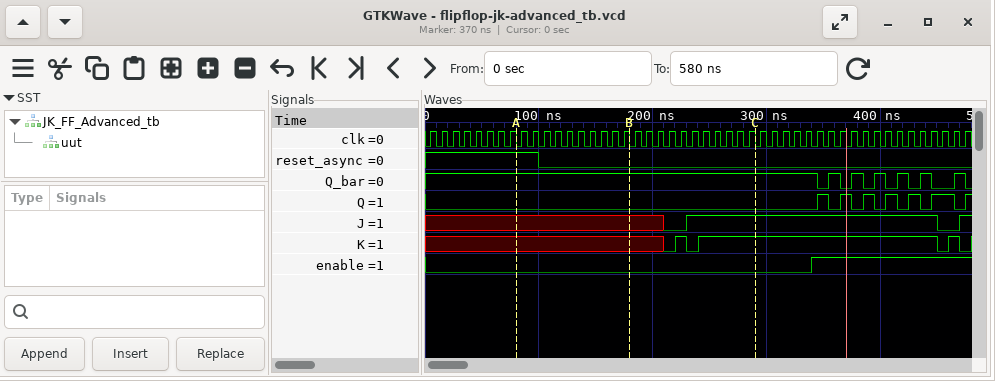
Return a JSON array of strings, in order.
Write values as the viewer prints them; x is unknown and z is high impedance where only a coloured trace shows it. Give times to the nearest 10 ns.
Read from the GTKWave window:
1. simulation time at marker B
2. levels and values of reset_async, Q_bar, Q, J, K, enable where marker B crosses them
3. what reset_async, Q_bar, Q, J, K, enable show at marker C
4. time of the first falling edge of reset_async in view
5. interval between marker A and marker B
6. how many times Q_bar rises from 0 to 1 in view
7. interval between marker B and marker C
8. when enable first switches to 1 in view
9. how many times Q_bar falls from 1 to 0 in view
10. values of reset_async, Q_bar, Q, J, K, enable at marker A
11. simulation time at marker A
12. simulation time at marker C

["180 ns", "reset_async=0, Q_bar=1, Q=0, J=x, K=x, enable=0", "reset_async=0, Q_bar=1, Q=0, J=1, K=1, enable=0", "100 ns", "100 ns", "6", "110 ns", "340 ns", "7", "reset_async=1, Q_bar=1, Q=0, J=x, K=x, enable=0", "80 ns", "290 ns"]
